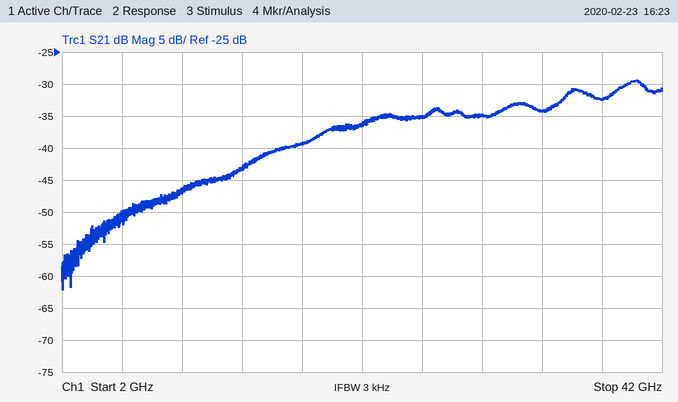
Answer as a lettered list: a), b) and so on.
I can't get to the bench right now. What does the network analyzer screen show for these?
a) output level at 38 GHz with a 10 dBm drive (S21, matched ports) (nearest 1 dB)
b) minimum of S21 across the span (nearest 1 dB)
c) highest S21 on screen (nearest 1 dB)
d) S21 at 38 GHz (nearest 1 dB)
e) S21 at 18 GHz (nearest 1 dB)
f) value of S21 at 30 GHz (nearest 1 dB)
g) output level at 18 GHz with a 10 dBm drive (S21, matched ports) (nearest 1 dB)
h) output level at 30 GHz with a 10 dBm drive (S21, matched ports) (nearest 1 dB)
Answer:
a) -22 dBm
b) -62 dB
c) -29 dB
d) -32 dB
e) -39 dB
f) -35 dB
g) -29 dBm
h) -25 dBm
